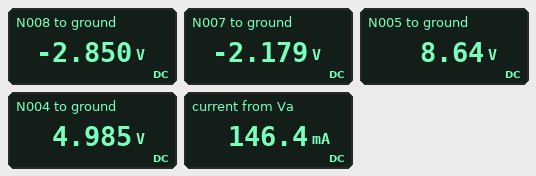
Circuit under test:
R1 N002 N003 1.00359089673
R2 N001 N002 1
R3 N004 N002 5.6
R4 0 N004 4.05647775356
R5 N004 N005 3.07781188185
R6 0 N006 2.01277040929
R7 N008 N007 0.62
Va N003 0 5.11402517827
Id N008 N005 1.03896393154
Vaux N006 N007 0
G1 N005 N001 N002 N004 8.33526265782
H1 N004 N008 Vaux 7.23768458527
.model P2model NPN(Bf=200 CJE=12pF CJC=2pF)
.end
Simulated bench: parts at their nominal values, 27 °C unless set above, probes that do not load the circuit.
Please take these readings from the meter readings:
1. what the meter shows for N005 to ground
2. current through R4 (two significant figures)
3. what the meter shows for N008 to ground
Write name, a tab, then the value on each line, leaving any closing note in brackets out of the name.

what the meter shows for N005 to ground	8.64 V
current through R4	1.2 A
what the meter shows for N008 to ground	-2.850 V
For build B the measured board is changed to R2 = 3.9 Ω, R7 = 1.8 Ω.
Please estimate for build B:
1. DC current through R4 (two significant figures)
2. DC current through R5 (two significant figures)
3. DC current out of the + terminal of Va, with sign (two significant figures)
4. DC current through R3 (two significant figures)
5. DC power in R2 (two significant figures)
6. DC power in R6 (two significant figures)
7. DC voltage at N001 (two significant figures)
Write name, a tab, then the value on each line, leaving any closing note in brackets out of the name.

DC current through R4	1.3 A
DC current through R5	790 mA
DC current out of the + terminal of Va, with sign	-240 mA
DC current through R3	5.3 mA
DC power in R2	240 mW
DC power in R6	4.9 W
DC voltage at N001	6.3 V
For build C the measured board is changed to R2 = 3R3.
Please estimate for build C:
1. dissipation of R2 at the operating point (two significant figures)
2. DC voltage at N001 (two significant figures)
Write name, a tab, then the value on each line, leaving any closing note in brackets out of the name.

dissipation of R2 at the operating point	74 mW
DC voltage at N001	4.5 V
